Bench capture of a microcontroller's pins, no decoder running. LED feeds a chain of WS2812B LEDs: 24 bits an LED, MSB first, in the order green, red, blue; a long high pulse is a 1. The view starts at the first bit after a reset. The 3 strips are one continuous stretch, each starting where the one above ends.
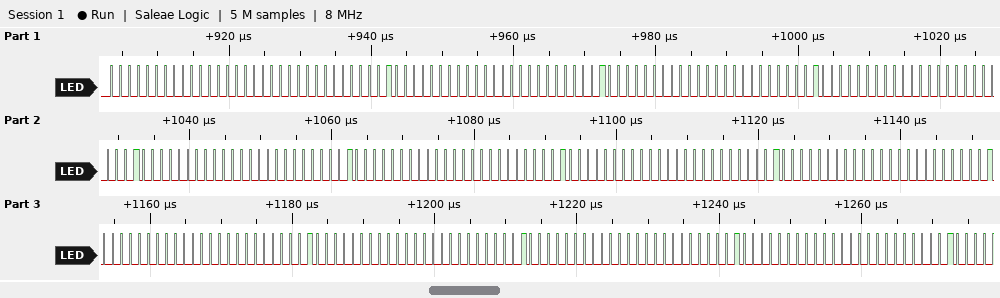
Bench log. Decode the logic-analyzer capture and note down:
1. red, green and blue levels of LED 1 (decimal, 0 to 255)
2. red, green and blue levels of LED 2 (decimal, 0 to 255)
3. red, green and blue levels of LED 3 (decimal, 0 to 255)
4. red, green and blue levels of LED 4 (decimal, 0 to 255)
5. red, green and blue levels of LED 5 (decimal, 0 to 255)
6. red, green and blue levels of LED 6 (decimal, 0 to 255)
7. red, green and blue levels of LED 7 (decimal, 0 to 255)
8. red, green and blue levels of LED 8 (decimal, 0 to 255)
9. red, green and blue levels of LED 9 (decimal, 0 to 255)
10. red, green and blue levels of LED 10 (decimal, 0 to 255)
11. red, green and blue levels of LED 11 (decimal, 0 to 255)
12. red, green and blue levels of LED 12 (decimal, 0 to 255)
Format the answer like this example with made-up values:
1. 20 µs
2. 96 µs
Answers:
1. 0, 0, 0
2. 0, 1, 0
3. 0, 1, 0
4. 0, 1, 0
5. 0, 1, 0
6. 0, 1, 0
7. 0, 1, 0
8. 0, 1, 0
9. 0, 1, 0
10. 0, 1, 0
11. 0, 1, 0
12. 0, 1, 0
